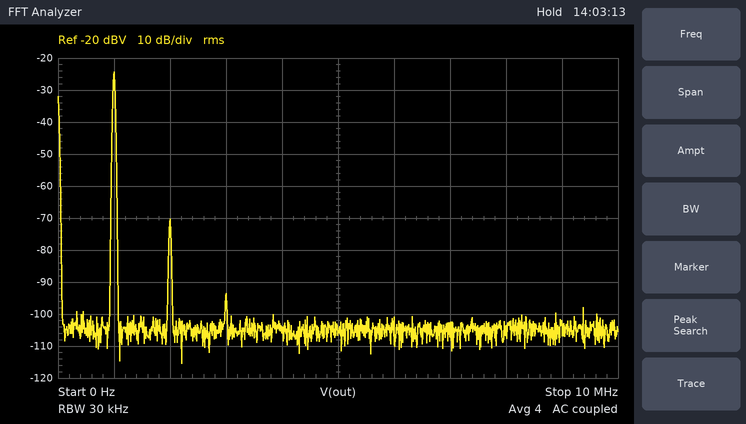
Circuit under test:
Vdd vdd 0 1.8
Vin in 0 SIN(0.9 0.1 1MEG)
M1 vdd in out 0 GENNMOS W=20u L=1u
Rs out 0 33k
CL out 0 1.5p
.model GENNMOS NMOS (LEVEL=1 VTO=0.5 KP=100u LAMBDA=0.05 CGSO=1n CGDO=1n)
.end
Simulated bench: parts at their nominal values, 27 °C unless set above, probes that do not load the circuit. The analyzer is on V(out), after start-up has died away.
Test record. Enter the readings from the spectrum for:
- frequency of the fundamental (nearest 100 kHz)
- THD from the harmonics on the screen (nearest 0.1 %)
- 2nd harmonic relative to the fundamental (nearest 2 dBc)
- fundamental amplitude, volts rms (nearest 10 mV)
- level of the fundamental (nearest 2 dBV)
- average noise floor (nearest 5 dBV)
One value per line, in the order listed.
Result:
1.0 MHz
0.5 %
-46 dBc
60 mV
-24 dBV
-105 dBV
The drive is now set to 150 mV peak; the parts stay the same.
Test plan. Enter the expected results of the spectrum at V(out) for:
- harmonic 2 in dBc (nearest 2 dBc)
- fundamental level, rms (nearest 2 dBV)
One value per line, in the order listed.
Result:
-42 dBc
-20 dBV
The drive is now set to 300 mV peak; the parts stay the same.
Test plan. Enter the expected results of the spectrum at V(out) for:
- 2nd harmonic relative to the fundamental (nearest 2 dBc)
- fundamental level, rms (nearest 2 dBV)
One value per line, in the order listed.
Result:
-34 dBc
-14 dBV
